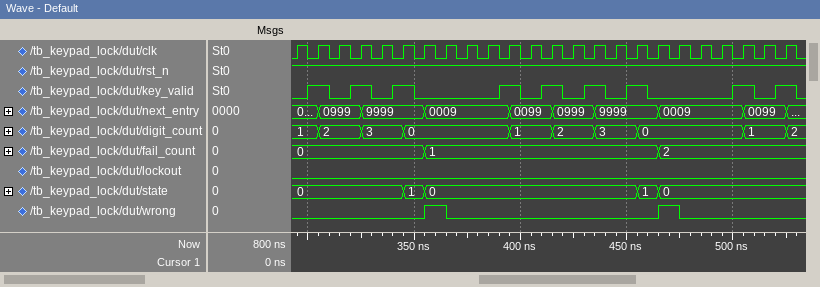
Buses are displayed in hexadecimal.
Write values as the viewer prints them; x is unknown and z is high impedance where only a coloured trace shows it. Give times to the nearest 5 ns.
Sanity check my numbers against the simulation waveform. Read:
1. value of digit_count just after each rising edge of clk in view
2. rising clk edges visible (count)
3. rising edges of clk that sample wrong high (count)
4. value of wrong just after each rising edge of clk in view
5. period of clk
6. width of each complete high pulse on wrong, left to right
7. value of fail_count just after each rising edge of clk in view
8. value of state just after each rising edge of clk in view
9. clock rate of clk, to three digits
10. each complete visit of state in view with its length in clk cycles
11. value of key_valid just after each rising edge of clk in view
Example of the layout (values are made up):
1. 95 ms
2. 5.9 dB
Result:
1. 1, 2, 2, 3, 3, 0, 0, 0, 0, 0, 1, 1, 2, 2, 3, 3, 0, 0, 0, 0, 0, 1, 1, 2
2. 24
3. 2
4. 0 0 0 0 0 0 1 0 0 0 0 0 0 0 0 0 0 1 0 0 0 0 0 0
5. 10 ns
6. 10 ns, 10 ns
7. 0, 0, 0, 0, 0, 0, 1, 1, 1, 1, 1, 1, 1, 1, 1, 1, 1, 2, 2, 2, 2, 2, 2, 2
8. 0, 0, 0, 0, 0, 1, 0, 0, 0, 0, 0, 0, 0, 0, 0, 0, 1, 0, 0, 0, 0, 0, 0, 0
9. 100 MHz
10. 1: 1, 0: 10, 1: 1
11. 0 1 0 1 0 1 0 0 0 0 1 0 1 0 1 0 1 0 0 0 0 1 0 1
